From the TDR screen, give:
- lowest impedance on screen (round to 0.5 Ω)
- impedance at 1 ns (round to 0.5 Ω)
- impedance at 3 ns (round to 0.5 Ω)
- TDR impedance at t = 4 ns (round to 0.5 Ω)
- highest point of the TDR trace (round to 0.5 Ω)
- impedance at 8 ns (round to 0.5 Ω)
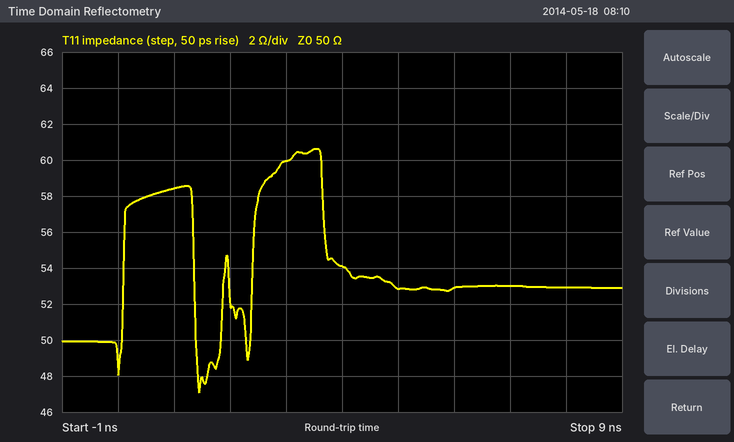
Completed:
47.0 Ω
58.5 Ω
60.0 Ω
54.0 Ω
60.5 Ω
53.0 Ω
